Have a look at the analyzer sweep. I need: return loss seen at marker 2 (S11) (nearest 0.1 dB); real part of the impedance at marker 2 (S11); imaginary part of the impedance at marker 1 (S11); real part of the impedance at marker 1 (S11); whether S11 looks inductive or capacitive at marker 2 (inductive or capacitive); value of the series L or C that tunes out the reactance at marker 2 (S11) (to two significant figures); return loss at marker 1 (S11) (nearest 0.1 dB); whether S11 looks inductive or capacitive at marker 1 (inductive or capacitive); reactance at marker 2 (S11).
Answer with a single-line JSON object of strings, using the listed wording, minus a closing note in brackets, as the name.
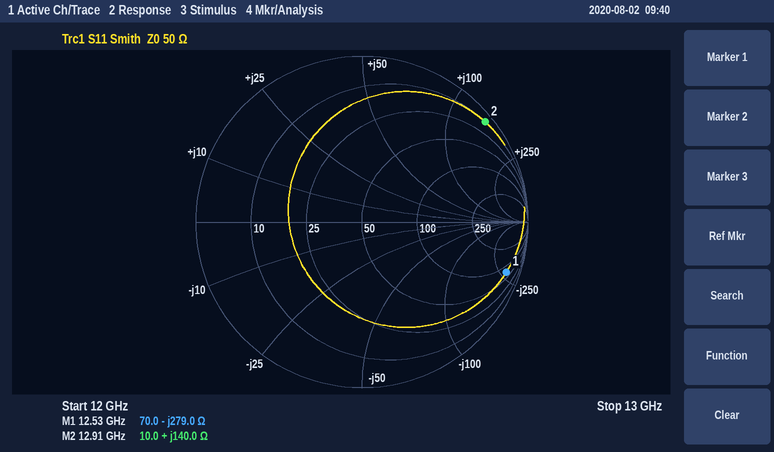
{"return loss seen at marker 2 (S11)": "0.4 dB", "real part of the impedance at marker 2": "10.0 Ω", "imaginary part of the impedance at marker 1": "-279.0 Ω", "real part of the impedance at marker 1": "70.0 Ω", "whether S11 looks inductive or capacitive at marker 2": "inductive", "value of the series L or C that tunes out the reactance at marker 2 (S11)": "88 fF", "return loss at marker 1 (S11)": "0.7 dB", "whether S11 looks inductive or capacitive at marker 1": "capacitive", "reactance at marker 2": "+140.0 Ω"}
